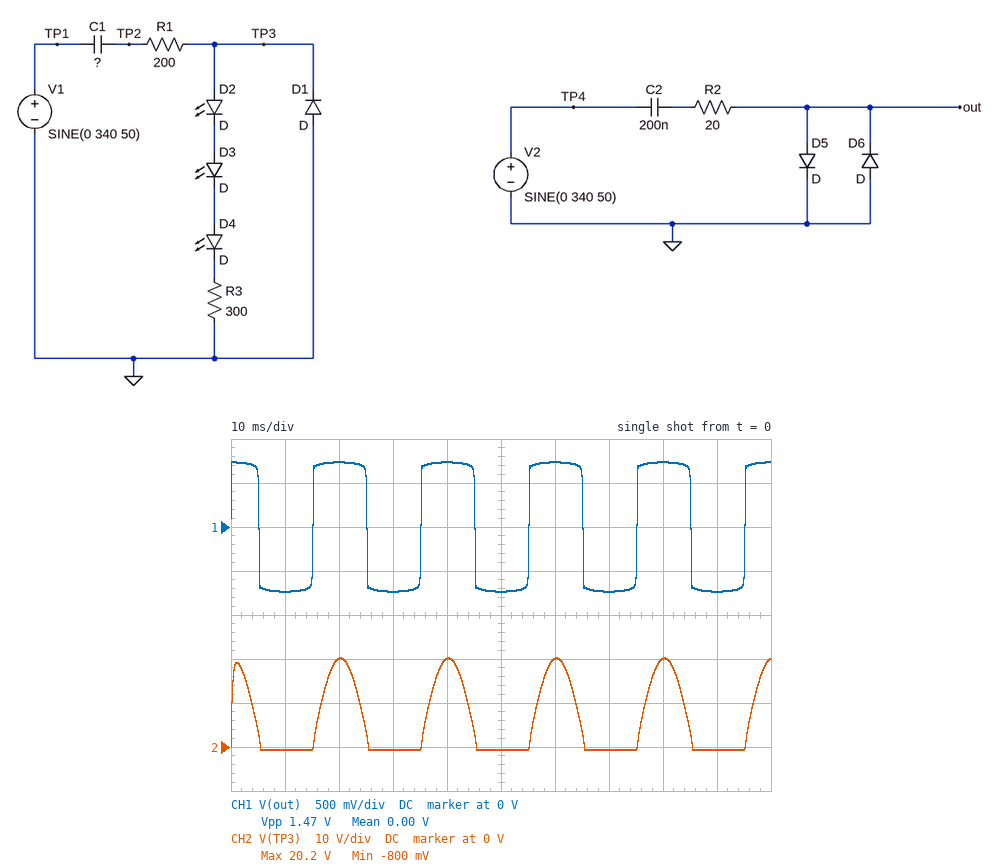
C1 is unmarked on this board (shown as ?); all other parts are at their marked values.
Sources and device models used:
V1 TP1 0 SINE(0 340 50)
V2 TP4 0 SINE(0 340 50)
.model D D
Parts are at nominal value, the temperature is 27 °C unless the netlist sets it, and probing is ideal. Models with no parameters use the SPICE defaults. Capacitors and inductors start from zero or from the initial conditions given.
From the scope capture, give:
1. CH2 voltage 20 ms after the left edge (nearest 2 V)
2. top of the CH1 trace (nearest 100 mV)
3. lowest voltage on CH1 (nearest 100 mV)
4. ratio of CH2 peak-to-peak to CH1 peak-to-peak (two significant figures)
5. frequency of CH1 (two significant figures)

20 V
700 mV
-700 mV
14
50 Hz
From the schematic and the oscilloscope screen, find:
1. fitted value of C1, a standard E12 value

560 nF
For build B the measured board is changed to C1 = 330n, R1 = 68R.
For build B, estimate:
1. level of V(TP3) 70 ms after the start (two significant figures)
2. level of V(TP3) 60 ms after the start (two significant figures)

-750 mV
13 V
